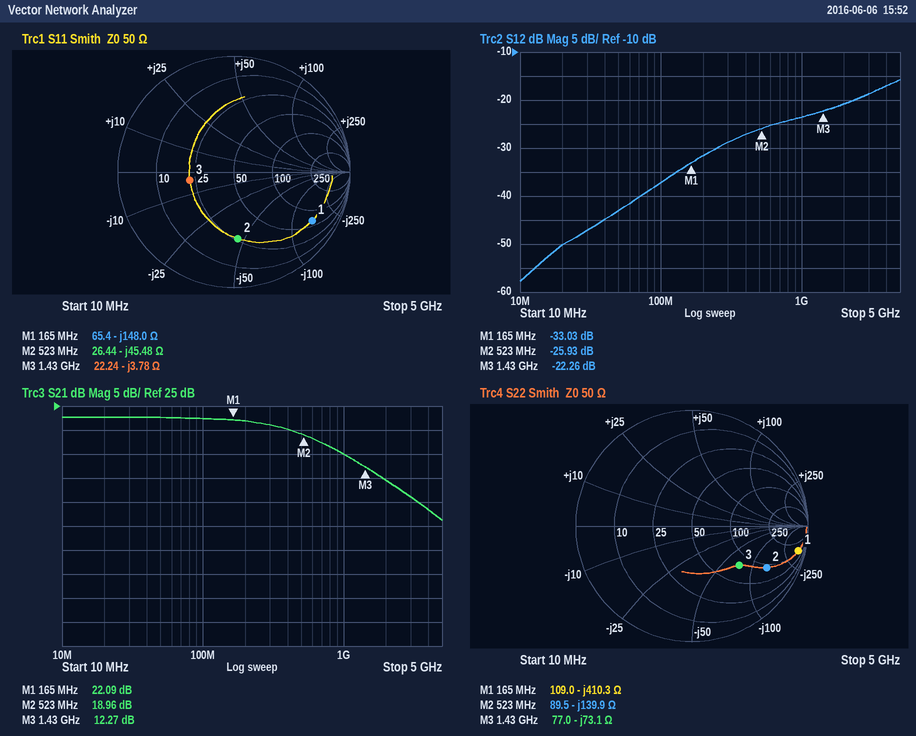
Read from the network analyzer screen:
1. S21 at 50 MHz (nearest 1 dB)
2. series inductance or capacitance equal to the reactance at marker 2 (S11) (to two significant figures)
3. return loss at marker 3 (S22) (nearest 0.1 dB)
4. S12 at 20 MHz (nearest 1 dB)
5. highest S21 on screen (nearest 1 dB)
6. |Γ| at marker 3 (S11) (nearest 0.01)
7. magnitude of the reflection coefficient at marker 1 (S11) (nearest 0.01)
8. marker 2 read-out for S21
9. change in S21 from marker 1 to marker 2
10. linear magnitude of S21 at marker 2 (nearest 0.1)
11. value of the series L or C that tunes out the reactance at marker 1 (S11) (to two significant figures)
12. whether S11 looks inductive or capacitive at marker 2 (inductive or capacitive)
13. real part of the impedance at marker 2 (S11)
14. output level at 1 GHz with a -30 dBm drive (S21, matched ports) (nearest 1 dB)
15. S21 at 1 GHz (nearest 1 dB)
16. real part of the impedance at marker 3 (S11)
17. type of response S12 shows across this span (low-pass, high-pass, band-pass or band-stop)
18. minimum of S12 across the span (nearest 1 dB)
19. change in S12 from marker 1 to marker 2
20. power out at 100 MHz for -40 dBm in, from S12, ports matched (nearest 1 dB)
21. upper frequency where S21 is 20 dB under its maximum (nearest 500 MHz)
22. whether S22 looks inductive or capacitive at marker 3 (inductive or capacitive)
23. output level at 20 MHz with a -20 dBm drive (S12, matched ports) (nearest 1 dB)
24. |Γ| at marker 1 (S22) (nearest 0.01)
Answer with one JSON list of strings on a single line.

["23 dB", "6.7 pF", "5.5 dB", "-50 dB", "23 dB", "0.39", "0.79", "18.96 dB", "-3.13 dB", "8.9", "140 nH", "capacitive", "26.44 Ω", "-15 dBm", "15 dB", "22.24 Ω", "high-pass", "-58 dB", "7.10 dB", "-77 dBm", "4.5 GHz", "capacitive", "-70 dBm", "0.94"]
